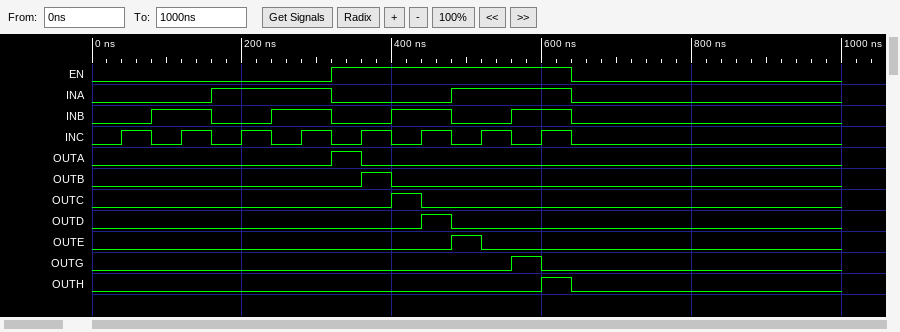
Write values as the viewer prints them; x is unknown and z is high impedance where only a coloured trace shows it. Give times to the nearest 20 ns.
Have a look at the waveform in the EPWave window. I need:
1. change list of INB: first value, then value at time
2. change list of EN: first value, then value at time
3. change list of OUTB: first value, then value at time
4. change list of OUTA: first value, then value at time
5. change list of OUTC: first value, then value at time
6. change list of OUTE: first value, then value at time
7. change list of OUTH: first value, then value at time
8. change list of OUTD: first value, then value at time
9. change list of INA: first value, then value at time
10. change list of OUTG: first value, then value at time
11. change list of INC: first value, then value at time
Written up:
0, 1 at 80 ns, 0 at 160 ns, 1 at 240 ns, 0 at 320 ns, 1 at 400 ns, 0 at 480 ns, 1 at 560 ns, 0 at 640 ns
0, 1 at 320 ns, 0 at 640 ns
0, 1 at 360 ns, 0 at 400 ns
0, 1 at 320 ns, 0 at 360 ns
0, 1 at 400 ns, 0 at 440 ns
0, 1 at 480 ns, 0 at 520 ns
0, 1 at 600 ns, 0 at 640 ns
0, 1 at 440 ns, 0 at 480 ns
0, 1 at 160 ns, 0 at 320 ns, 1 at 480 ns, 0 at 640 ns
0, 1 at 560 ns, 0 at 600 ns
0, 1 at 40 ns, 0 at 80 ns, 1 at 120 ns, 0 at 160 ns, 1 at 200 ns, 0 at 240 ns, 1 at 280 ns, 0 at 320 ns, 1 at 360 ns, 0 at 400 ns, 1 at 440 ns, 0 at 480 ns, 1 at 520 ns, 0 at 560 ns, 1 at 600 ns, 0 at 640 ns
